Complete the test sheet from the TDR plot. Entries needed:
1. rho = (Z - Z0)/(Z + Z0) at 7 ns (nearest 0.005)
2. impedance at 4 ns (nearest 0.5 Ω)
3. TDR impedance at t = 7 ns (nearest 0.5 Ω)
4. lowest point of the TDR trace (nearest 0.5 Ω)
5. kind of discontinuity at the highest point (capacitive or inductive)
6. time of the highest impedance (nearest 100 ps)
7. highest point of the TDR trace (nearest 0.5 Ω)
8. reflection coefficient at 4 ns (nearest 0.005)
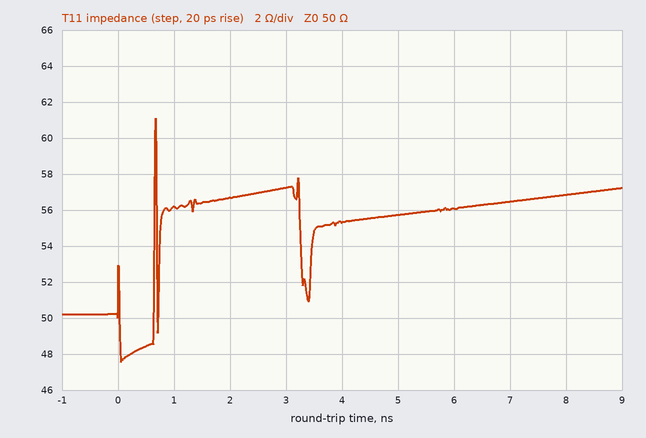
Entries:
+0.060
55.5 Ω
56.5 Ω
47.5 Ω
inductive
700 ps
61.0 Ω
+0.050
